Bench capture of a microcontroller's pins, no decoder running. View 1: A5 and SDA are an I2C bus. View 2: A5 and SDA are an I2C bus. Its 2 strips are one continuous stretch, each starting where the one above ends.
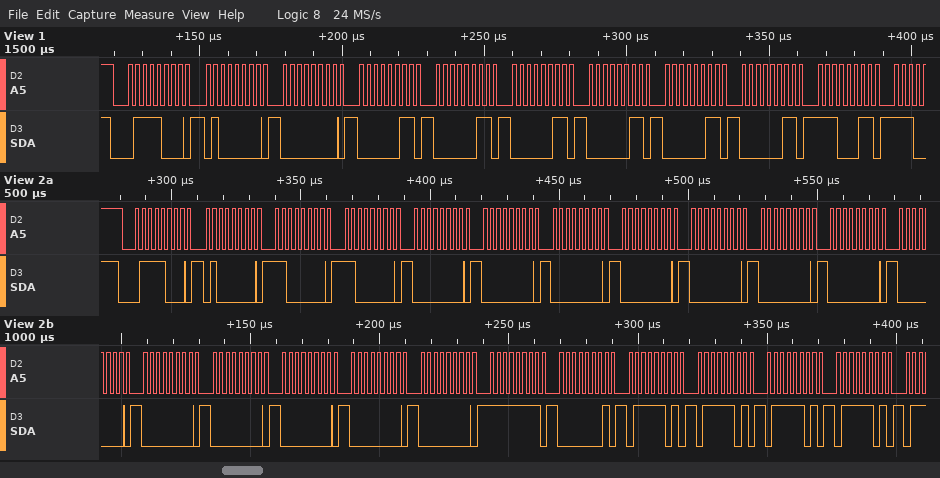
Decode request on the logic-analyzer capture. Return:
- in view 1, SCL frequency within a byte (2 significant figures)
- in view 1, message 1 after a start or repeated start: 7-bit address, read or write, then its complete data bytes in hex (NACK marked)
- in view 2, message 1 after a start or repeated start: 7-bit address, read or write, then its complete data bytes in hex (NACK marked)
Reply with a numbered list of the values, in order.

1. 400 kHz
2. 0x3C write: 40 00 03 03 03 03 03 03 E3
3. 0x3C write: 40 C0 C0 00 00 00 00 00 00 00 00 00 00 00 00 00 FF 01 7D 7D 7D 7D
